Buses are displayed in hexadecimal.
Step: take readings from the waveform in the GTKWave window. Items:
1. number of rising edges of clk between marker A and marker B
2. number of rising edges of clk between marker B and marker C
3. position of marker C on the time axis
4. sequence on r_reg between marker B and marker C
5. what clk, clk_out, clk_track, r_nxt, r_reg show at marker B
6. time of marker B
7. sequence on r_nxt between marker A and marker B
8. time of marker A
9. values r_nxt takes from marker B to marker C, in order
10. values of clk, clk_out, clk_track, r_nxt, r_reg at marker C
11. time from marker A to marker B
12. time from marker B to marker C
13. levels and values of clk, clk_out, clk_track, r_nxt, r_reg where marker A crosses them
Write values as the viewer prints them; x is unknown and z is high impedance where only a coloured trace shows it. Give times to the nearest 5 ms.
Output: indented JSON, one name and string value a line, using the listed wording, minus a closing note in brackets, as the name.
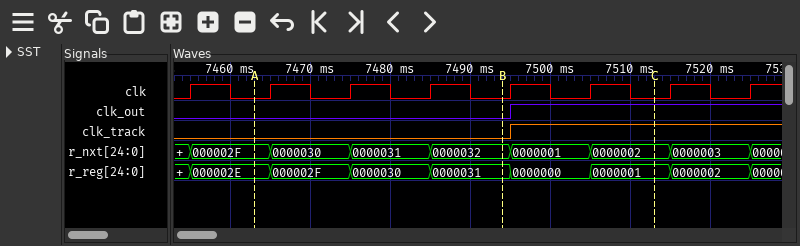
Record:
{
  "number of rising edges of clk between marker A and marker B": "3",
  "number of rising edges of clk between marker B and marker C": "2",
  "position of marker C on the time axis": "7515 ms",
  "sequence on r_reg between marker B and marker C": "0000031, 0000000, 0000001",
  "what clk, clk_out, clk_track, r_nxt, r_reg show at marker B": "clk=0, clk_out=0, clk_track=0, r_nxt=0000032, r_reg=0000031",
  "time of marker B": "7495 ms",
  "sequence on r_nxt between marker A and marker B": "000002F, 0000030, 0000031, 0000032",
  "time of marker A": "7465 ms",
  "values r_nxt takes from marker B to marker C, in order": "0000032, 0000001, 0000002",
  "values of clk, clk_out, clk_track, r_nxt, r_reg at marker C": "clk=0, clk_out=1, clk_track=1, r_nxt=0000002, r_reg=0000001",
  "time from marker A to marker B": "30 ms",
  "time from marker B to marker C": "20 ms",
  "levels and values of clk, clk_out, clk_track, r_nxt, r_reg where marker A crosses them": "clk=0, clk_out=0, clk_track=0, r_nxt=000002F, r_reg=000002E"
}
